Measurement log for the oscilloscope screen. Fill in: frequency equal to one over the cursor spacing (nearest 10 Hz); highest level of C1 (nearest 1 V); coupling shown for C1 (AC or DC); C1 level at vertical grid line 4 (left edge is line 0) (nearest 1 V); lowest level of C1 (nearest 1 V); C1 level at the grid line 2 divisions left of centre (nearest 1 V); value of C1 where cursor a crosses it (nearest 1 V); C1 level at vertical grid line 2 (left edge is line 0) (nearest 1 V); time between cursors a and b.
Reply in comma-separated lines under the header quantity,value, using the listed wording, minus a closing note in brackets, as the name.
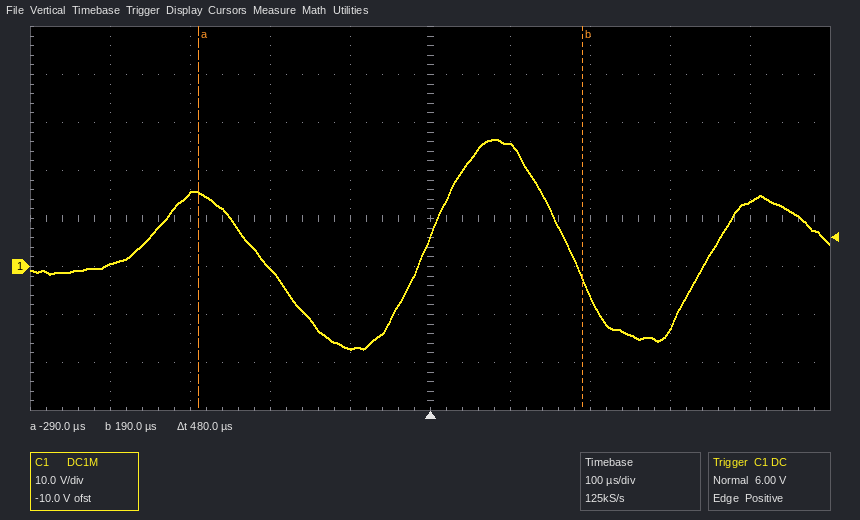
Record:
quantity,value
frequency equal to one over the cursor spacing,2.08 kHz
highest level of C1,26 V
coupling shown for C1,DC
C1 level at vertical grid line 4 (left edge is line 0),-17 V
lowest level of C1,-17 V
C1 level at the grid line 2 divisions left of centre,0 V
value of C1 where cursor a crosses it,15 V
C1 level at vertical grid line 2 (left edge is line 0),15 V
time between cursors a and b,480 µs
